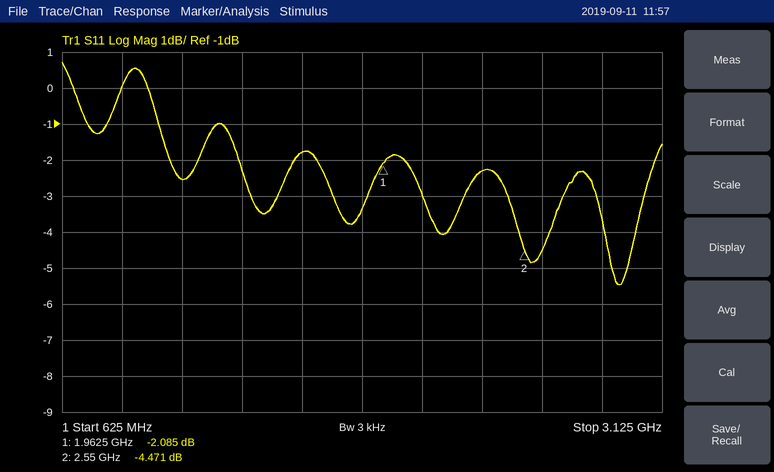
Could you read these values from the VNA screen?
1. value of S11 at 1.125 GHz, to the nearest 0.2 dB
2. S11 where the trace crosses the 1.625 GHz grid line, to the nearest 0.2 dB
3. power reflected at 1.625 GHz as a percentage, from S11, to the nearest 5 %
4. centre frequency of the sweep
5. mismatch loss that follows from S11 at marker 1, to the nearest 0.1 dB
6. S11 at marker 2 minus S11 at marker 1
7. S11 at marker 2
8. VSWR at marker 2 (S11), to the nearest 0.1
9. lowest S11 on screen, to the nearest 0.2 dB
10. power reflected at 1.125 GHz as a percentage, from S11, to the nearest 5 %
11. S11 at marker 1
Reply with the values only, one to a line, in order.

-2.6 dB
-1.8 dB
65 %
1.875 GHz
4.2 dB
-2.386 dB
-4.471 dB
4.0
-5.4 dB
55 %
-2.085 dB
